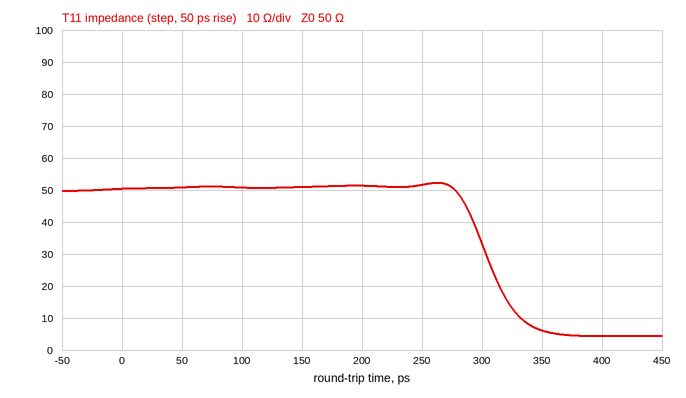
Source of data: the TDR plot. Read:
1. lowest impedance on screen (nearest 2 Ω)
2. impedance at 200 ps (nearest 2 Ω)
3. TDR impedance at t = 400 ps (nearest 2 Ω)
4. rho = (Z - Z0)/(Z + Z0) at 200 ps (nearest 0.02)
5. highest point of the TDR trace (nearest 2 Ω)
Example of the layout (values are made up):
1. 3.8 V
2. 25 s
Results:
1. 4 Ω
2. 52 Ω
3. 4 Ω
4. +0.02
5. 52 Ω
